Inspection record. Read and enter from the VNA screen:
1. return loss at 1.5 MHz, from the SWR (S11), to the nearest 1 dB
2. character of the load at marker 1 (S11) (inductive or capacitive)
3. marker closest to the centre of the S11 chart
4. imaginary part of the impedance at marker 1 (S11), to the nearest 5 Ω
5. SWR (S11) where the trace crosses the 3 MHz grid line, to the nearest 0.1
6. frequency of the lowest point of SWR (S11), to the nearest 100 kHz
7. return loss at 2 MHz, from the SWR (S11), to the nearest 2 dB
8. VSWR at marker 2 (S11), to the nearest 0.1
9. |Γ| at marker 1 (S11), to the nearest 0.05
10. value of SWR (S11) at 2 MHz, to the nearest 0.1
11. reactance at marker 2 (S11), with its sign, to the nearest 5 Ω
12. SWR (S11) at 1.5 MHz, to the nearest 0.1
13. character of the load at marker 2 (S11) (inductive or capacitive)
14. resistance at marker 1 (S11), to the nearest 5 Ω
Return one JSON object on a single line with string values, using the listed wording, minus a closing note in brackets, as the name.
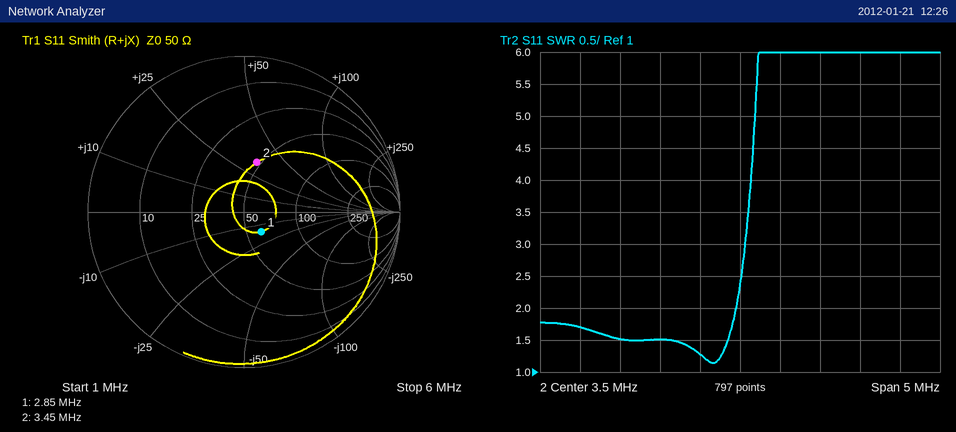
{"return loss at 1.5 MHz, from the SWR (S11), to the nearest 1 dB": "12 dB", "character of the load at marker 1 (S11)": "capacitive", "marker closest to the centre of the S11 chart": "marker 1", "imaginary part of the impedance at marker 1 (S11), to the nearest 5 Ω": "-15 Ω", "SWR (S11) where the trace crosses the 3 MHz grid line, to the nearest 0.1": "1.3", "frequency of the lowest point of SWR (S11), to the nearest 100 kHz": "3.2 MHz", "return loss at 2 MHz, from the SWR (S11), to the nearest 2 dB": "14 dB", "VSWR at marker 2 (S11), to the nearest 0.1": "2.0", "|Γ| at marker 1 (S11), to the nearest 0.05": "0.15", "value of SWR (S11) at 2 MHz, to the nearest 0.1": "1.5", "reactance at marker 2 (S11), with its sign, to the nearest 5 Ω": "+35 Ω", "SWR (S11) at 1.5 MHz, to the nearest 0.1": "1.7", "character of the load at marker 2 (S11)": "inductive", "resistance at marker 1 (S11), to the nearest 5 Ω": "60 Ω"}
